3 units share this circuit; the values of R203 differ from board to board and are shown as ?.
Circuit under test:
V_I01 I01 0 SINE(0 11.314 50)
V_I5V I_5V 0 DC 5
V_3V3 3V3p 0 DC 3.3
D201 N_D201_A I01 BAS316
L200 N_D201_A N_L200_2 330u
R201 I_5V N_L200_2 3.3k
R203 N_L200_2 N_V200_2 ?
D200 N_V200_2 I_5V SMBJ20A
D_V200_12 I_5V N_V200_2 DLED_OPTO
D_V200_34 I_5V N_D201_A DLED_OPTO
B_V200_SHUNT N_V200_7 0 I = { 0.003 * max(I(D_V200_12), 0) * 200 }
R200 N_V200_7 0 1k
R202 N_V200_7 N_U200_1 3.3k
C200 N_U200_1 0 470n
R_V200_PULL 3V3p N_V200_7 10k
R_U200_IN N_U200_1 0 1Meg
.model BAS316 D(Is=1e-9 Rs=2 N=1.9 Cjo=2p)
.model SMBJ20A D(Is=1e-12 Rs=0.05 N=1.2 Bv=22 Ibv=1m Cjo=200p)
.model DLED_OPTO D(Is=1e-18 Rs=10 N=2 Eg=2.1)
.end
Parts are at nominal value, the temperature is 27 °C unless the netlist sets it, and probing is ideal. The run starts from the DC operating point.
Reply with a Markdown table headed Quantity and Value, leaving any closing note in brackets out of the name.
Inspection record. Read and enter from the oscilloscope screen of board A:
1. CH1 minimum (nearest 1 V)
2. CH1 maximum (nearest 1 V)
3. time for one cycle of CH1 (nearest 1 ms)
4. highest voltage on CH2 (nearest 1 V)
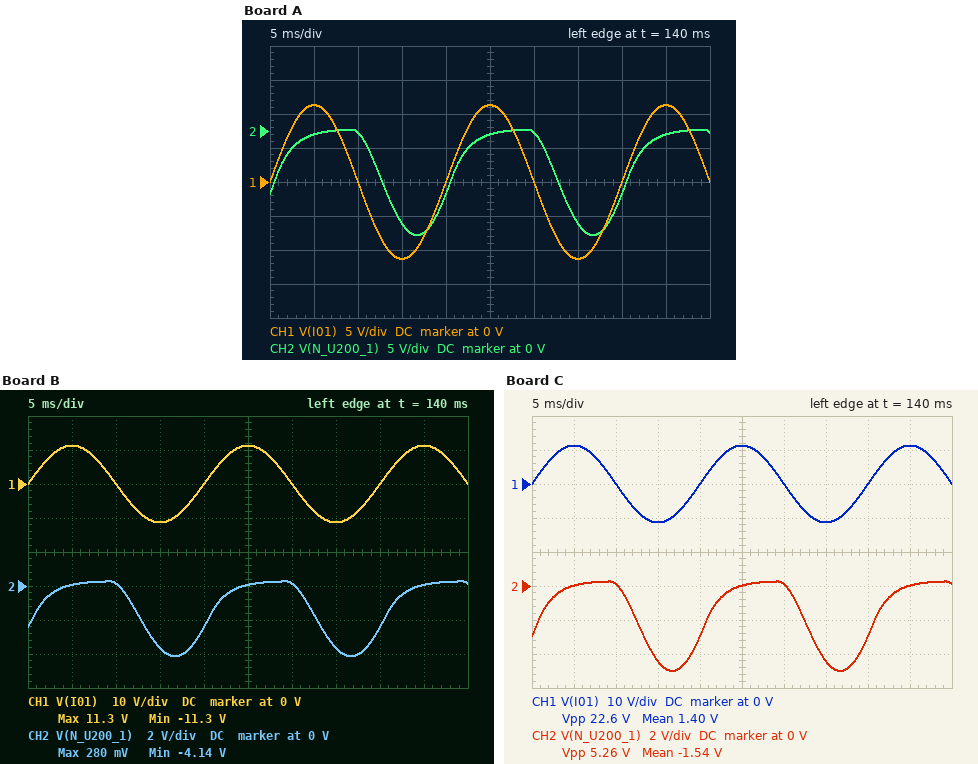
| Quantity | Value |
|---|---|
| CH1 minimum | -11 V |
| CH1 maximum | 11 V |
| time for one cycle of CH1 | 20 ms |
| highest voltage on CH2 | 0 V |
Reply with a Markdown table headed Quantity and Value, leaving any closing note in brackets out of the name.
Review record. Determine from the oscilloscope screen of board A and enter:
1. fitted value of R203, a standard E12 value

| Quantity | Value |
|---|---|
| fitted value of R203, a standard E12 value | 330 Ω |
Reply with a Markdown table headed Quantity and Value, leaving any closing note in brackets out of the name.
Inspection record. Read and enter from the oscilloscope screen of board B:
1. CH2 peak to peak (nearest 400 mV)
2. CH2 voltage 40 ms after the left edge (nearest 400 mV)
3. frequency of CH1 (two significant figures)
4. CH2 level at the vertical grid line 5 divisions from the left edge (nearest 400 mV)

| Quantity | Value |
|---|---|
| CH2 peak to peak | 4.4 V |
| CH2 voltage 40 ms after the left edge | -2.4 V |
| frequency of CH1 | 50 Hz |
| CH2 level at the vertical grid line 5 divisions from the left edge | 0 V |
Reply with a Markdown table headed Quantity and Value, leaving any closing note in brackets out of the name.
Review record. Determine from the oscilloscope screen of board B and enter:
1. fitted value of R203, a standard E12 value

| Quantity | Value |
|---|---|
| fitted value of R203, a standard E12 value | 1.2 kΩ |
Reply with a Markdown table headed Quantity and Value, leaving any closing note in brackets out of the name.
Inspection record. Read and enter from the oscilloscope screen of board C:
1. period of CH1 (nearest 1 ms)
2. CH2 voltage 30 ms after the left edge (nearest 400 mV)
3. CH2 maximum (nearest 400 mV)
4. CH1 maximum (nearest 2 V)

| Quantity | Value |
|---|---|
| period of CH1 | 20 ms |
| CH2 voltage 30 ms after the left edge | 0 V |
| CH2 maximum | 400 mV |
| CH1 maximum | 12 V |
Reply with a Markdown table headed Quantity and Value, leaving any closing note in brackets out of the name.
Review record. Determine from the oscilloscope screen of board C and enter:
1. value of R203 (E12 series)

| Quantity | Value |
|---|---|
| value of R203 | 1 kΩ |
